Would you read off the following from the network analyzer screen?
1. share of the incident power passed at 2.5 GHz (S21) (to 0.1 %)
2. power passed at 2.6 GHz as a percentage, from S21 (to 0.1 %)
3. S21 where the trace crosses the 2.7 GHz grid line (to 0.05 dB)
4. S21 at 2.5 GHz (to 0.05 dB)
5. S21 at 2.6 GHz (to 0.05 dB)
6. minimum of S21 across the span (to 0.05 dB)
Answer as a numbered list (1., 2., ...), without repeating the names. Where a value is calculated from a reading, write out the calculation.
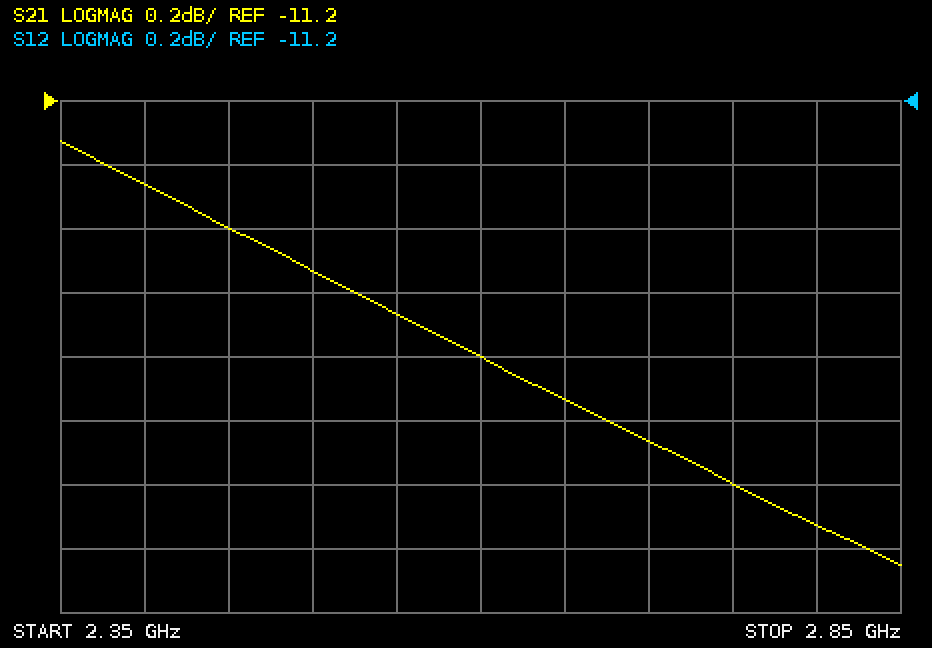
1. 10^(-11.75/10) ≈ 6.7 %
2. 10^(-12/10) ≈ 6.3 %
3. -12.25 dB
4. -11.75 dB
5. -12.00 dB
6. -12.65 dB
